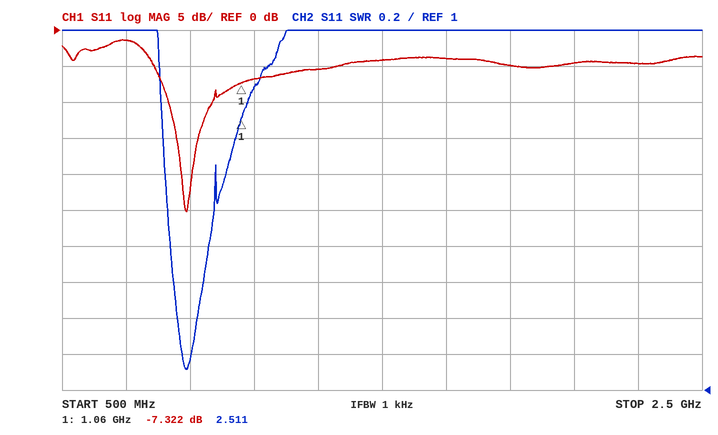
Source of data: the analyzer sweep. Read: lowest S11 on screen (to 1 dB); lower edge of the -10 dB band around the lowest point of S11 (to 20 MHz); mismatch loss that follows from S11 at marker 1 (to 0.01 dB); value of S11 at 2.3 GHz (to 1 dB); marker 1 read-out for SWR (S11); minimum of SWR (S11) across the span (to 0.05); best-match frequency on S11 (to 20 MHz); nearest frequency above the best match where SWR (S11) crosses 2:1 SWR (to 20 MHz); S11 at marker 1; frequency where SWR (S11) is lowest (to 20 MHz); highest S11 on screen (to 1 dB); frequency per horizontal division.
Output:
-25 dB
840 MHz
0.89 dB
-5 dB
2.511
1.10
880 MHz
980 MHz
-7.322 dB
880 MHz
-1 dB
200 MHz
